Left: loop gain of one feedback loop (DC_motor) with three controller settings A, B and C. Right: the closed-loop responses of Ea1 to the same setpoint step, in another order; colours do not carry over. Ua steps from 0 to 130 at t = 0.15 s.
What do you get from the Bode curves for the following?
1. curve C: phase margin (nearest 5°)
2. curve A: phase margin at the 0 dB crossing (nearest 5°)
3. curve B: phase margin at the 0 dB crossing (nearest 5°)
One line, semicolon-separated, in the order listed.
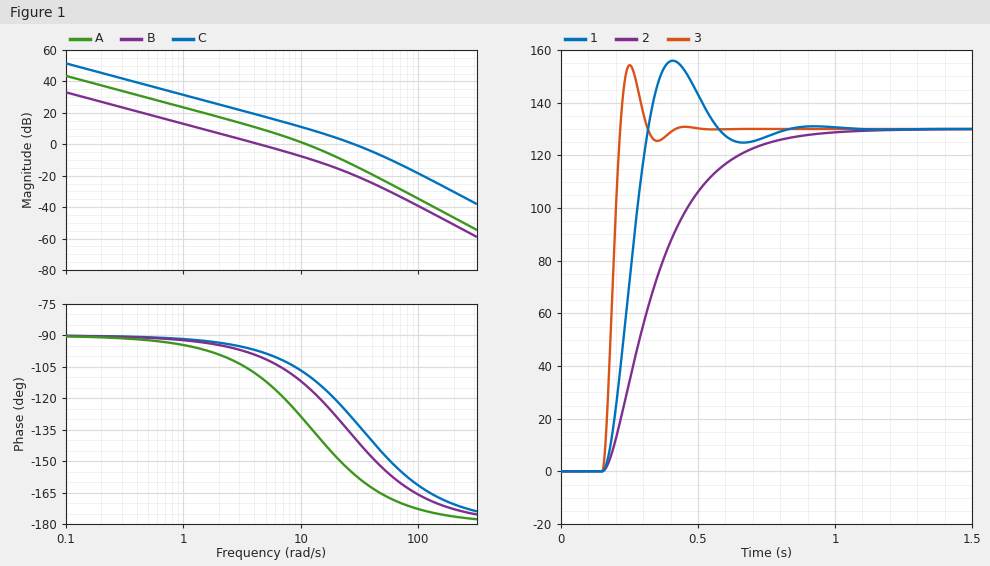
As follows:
50°; 50°; 80°
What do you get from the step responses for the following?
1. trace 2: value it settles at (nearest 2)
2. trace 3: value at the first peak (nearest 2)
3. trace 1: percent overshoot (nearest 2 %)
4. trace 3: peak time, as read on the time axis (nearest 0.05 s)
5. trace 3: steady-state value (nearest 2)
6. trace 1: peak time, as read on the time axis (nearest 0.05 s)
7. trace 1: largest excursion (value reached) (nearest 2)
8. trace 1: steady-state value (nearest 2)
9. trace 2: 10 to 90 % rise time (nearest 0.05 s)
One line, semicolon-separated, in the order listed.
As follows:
130; 154; 20 %; 0.25 s; 130; 0.40 s; 156; 130; 0.40 s
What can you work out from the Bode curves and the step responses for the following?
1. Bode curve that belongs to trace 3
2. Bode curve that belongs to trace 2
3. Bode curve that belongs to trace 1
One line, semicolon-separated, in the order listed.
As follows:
C; B; A
